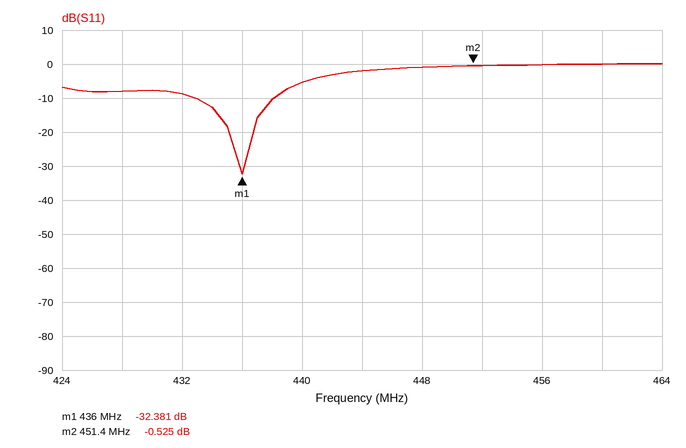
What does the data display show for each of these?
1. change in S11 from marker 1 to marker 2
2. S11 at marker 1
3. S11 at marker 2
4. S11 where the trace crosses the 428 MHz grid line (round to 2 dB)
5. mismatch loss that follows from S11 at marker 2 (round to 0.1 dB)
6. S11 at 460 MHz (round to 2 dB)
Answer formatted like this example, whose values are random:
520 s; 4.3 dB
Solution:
31.856 dB; -32.381 dB; -0.525 dB; -8 dB; 9.4 dB; 0 dB
